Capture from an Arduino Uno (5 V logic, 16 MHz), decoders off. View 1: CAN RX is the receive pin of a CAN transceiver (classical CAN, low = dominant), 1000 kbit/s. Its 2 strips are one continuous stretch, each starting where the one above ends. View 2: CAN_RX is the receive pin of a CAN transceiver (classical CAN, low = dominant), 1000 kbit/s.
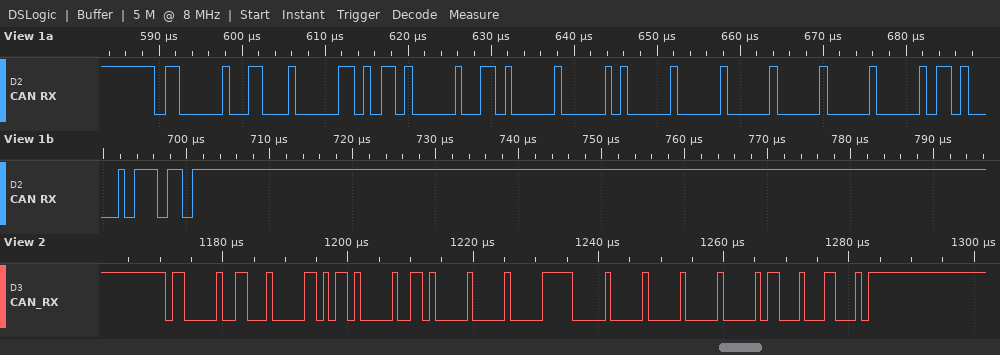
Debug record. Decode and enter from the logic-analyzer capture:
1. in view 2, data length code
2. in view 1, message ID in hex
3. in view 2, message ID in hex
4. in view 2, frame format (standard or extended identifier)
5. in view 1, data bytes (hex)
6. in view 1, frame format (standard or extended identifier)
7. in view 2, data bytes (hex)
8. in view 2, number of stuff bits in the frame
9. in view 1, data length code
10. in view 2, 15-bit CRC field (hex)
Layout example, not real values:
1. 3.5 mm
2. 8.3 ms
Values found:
1. 8
2. 0x603
3. 0x603
4. standard
5. 2B 40 68 00 80 00 00 00
6. standard
7. 2B 40 68 00 0F 00 00 00
8. 12
9. 8
10. 0x3118
